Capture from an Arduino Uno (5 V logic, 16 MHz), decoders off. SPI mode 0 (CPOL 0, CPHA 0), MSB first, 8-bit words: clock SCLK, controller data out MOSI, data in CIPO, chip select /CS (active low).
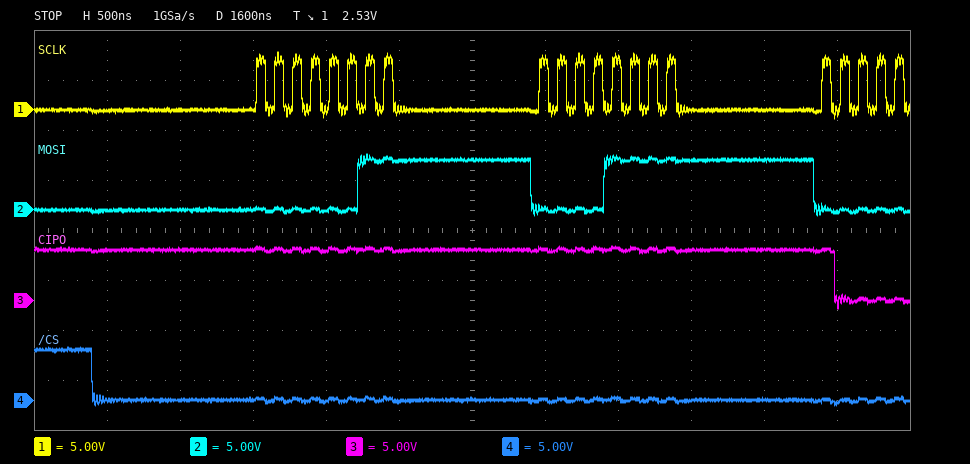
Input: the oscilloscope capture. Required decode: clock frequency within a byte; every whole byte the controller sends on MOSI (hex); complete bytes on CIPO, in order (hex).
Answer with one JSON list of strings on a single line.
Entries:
["8 MHz", "03 0F", "FF FF"]
